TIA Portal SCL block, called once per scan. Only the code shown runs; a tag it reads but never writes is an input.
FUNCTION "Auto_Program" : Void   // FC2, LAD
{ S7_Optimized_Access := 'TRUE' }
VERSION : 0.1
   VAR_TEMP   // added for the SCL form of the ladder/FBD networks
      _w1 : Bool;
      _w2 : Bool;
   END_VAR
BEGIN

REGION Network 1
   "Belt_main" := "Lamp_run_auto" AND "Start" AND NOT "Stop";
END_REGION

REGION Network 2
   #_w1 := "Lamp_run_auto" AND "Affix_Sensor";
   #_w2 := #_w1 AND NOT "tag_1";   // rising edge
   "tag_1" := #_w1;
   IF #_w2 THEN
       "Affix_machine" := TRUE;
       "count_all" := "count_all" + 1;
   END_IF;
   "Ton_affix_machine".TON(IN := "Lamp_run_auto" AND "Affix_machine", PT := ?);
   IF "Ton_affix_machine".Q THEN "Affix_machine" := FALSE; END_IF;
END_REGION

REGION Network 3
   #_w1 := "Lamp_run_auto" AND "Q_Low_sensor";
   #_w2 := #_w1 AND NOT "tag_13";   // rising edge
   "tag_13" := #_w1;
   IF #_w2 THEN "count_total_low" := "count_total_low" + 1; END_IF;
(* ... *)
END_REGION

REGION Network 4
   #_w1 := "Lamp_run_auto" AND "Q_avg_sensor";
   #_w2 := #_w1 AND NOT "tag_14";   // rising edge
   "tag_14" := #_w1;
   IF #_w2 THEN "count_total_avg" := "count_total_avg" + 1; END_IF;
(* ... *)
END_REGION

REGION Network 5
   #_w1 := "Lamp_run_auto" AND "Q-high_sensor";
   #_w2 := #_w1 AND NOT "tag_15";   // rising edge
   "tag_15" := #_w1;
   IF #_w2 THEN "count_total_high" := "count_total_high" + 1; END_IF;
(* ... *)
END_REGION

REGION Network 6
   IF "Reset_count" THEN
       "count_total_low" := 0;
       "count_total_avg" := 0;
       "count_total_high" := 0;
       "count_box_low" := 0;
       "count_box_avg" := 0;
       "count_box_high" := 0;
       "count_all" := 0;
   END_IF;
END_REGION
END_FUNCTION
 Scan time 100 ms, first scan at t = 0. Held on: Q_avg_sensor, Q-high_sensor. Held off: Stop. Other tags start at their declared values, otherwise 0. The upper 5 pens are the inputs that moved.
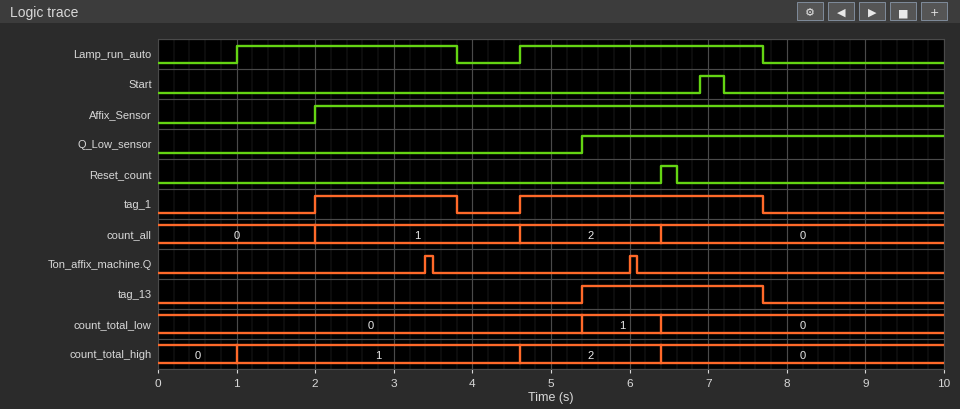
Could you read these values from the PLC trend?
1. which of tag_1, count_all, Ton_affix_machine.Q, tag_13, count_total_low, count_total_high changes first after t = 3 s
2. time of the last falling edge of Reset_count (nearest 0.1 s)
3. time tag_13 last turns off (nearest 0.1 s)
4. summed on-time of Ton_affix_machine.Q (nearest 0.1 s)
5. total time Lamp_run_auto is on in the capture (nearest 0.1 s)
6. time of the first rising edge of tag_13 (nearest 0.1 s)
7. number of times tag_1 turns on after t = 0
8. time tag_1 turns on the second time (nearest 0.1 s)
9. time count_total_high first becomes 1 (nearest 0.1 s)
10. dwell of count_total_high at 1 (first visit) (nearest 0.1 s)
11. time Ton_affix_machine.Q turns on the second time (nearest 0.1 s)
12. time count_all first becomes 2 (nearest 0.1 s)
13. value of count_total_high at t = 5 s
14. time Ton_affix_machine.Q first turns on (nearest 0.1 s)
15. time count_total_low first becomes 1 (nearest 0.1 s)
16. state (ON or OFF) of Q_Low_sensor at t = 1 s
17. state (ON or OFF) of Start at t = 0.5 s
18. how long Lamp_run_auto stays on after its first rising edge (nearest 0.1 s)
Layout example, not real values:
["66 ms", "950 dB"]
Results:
["Ton_affix_machine.Q", "6.6 s", "7.7 s", "0.2 s", "5.9 s", "5.4 s", "2", "4.6 s", "1.0 s", "3.6 s", "6.0 s", "4.6 s", "2", "3.4 s", "5.4 s", "OFF", "OFF", "2.8 s"]
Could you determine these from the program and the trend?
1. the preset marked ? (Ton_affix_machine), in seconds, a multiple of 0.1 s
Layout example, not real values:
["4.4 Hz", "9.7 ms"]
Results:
["1.4 s"]
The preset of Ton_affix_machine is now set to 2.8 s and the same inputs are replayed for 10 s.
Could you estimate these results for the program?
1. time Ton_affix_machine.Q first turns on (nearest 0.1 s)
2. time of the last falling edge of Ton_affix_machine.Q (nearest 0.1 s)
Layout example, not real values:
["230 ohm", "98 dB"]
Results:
["7.4 s", "7.5 s"]
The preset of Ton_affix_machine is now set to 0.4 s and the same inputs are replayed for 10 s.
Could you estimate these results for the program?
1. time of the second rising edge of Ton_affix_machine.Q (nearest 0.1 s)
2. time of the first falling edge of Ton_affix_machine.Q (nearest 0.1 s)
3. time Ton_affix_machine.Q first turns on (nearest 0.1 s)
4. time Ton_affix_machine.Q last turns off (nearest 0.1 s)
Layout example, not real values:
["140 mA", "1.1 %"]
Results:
["5.0 s", "2.5 s", "2.4 s", "5.1 s"]
